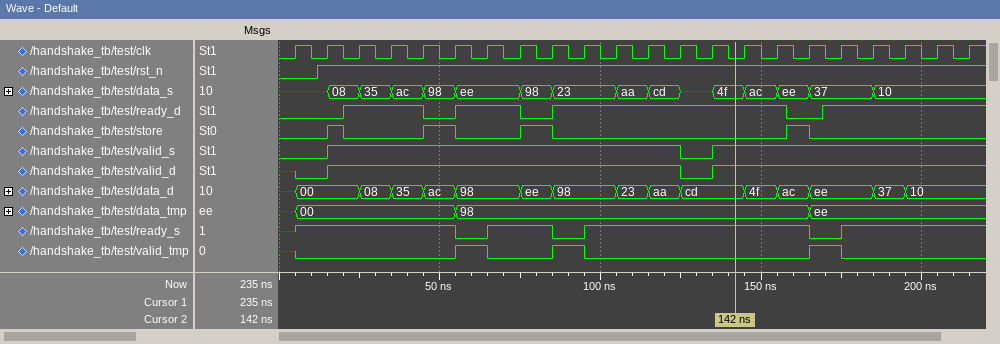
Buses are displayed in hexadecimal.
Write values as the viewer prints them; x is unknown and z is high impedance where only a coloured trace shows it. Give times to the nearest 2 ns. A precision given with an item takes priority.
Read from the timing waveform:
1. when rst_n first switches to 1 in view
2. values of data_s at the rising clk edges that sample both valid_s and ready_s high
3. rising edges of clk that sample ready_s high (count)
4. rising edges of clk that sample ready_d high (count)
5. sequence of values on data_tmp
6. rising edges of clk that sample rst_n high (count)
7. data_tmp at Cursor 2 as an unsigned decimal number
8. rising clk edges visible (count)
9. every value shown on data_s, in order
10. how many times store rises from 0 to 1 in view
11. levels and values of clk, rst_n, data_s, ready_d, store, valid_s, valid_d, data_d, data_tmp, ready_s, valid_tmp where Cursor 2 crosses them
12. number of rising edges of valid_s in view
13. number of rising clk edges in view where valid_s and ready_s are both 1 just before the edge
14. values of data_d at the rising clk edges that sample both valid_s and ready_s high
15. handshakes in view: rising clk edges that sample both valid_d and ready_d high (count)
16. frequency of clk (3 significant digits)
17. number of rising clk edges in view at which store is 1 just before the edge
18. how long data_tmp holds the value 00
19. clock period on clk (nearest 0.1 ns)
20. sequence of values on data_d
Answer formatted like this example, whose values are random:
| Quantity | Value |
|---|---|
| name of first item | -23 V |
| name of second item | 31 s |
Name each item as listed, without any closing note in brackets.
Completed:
| Quantity | Value |
|---|---|
| when rst_n first switches to 1 in view | 12 ns |
| values of data_s at the rising clk edges that sample both valid_s and ready_s high | 08, 35, ac, 98, ee, 98, 23, aa, cd, 4f, ac, ee, 37, 10, 10, 10 |
| rising edges of clk that sample ready_s high | 18 |
| rising edges of clk that sample ready_d high | 17 |
| sequence of values on data_tmp | x, 00, 98, ee |
| rising edges of clk that sample rst_n high | 21 |
| data_tmp at Cursor 2 as an unsigned decimal number | 152 |
| rising clk edges visible | 22 |
| every value shown on data_s, in order | x, 08, 35, ac, 98, ee, 98, 23, aa, cd, x, 4f, ac, ee, 37, 10 |
| how many times store rises from 0 to 1 in view | 4 |
| levels and values of clk, rst_n, data_s, ready_d, store, valid_s, valid_d, data_d, data_tmp, ready_s, valid_tmp where Cursor 2 crosses them | clk=0, rst_n=1, data_s=4f, ready_d=1, store=0, valid_s=1, valid_d=1, data_d=cd, data_tmp=98, ready_s=1, valid_tmp=0 |
| number of rising edges of valid_s in view | 2 |
| number of rising clk edges in view where valid_s and ready_s are both 1 just before the edge | 16 |
| values of data_d at the rising clk edges that sample both valid_s and ready_s high | 00, 08, 35, ac, 98, ee, 98, 23, aa, cd, 4f, ac, ee, 37, 10, 10 |
| handshakes in view: rising clk edges that sample both valid_d and ready_d high | 16 |
| frequency of clk | 100 MHz |
| number of rising clk edges in view at which store is 1 just before the edge | 3 |
| how long data_tmp holds the value 00 | 50 ns |
| clock period on clk | 10 ns |
| sequence of values on data_d | x, 00, 08, 35, ac, 98, ee, 98, 23, aa, cd, 4f, ac, ee, 37, 10 |
